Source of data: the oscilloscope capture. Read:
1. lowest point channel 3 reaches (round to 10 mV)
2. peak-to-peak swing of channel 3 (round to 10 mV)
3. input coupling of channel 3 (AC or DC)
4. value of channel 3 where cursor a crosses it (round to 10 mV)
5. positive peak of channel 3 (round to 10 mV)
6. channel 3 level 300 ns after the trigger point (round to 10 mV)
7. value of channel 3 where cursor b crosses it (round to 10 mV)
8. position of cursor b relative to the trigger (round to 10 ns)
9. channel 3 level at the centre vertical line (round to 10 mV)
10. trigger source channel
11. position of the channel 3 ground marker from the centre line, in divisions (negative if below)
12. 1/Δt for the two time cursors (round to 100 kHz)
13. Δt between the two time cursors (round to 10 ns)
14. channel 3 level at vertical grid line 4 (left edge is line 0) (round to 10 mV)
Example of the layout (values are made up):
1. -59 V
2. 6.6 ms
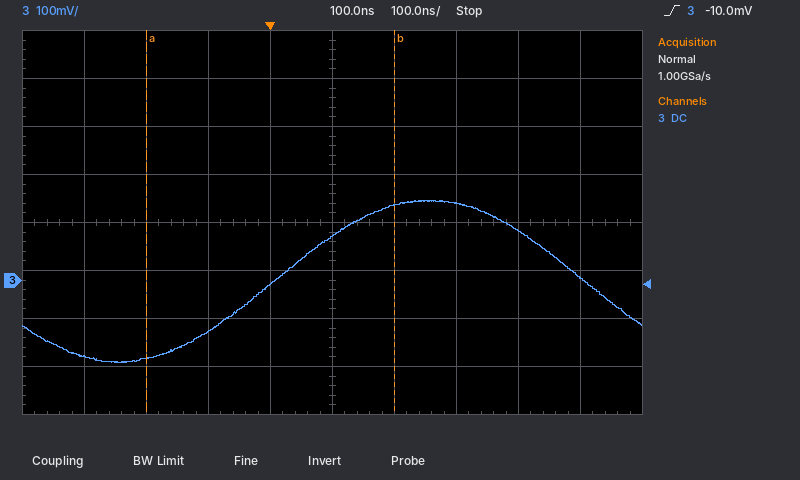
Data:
1. -170 mV
2. 340 mV
3. DC
4. -160 mV
5. 170 mV
6. 160 mV
7. 160 mV
8. +200 ns
9. 90 mV
10. channel 3
11. -1.2 div
12. 2.5 MHz
13. 400 ns
14. -10 mV
